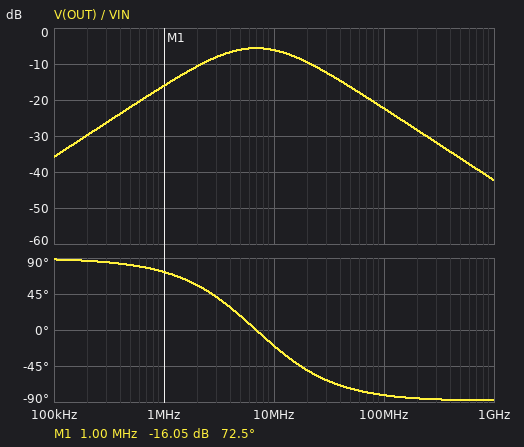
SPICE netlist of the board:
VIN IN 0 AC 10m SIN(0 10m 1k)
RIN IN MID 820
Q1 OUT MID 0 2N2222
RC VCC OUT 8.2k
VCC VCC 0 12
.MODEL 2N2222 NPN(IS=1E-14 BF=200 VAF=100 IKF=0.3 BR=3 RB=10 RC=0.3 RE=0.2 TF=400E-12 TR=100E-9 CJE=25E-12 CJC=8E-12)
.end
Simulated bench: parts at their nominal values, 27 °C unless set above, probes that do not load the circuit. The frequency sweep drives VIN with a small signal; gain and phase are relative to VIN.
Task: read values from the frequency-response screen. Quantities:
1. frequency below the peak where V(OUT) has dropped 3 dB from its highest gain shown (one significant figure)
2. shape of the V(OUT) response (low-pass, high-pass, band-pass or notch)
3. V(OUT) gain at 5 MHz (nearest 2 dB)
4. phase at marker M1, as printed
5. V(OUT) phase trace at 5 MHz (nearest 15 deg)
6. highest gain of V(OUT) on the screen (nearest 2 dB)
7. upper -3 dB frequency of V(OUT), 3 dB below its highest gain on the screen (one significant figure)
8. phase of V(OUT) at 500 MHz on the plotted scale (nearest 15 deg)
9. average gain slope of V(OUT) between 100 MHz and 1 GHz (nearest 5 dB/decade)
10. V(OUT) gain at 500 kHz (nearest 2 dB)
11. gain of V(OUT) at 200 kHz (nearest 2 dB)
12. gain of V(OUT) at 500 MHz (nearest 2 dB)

3 MHz
band-pass
-6 dB
72.5 deg
15 deg
-6 dB
20 MHz
-90 deg
-20 dB/decade
-22 dB
-30 dB
-36 dB
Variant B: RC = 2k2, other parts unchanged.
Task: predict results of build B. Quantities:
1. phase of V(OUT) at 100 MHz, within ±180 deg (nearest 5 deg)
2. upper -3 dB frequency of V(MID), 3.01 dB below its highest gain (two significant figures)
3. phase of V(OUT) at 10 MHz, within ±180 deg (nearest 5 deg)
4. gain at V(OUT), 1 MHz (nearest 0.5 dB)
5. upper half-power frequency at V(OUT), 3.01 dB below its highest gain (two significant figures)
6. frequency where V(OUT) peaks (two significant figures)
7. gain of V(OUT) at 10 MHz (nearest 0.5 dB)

-70 deg
6.7 MHz
15 deg
-27.5 dB
38 MHz
13 MHz
-13.0 dB
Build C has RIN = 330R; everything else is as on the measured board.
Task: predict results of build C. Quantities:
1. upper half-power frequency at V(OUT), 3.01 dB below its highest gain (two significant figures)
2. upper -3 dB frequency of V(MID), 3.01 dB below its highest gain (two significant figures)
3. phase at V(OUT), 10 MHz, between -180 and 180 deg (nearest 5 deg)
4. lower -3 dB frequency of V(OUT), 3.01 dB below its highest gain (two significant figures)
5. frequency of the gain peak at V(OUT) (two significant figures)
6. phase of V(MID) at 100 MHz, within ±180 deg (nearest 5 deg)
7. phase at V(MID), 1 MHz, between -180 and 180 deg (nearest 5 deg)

30 MHz
18 MHz
5 deg
3.9 MHz
11 MHz
-70 deg
-5 deg
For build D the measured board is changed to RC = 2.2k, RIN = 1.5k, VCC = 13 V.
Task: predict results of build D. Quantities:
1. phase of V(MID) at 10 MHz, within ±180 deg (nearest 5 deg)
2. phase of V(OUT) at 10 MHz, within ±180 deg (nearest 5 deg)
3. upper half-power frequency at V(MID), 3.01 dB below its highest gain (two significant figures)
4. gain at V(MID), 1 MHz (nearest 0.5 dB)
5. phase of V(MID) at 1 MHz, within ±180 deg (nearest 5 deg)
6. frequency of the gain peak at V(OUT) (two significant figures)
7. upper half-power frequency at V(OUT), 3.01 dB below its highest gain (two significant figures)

-65 deg
0 deg
3.7 MHz
-0.5 dB
-15 deg
10 MHz
34 MHz
